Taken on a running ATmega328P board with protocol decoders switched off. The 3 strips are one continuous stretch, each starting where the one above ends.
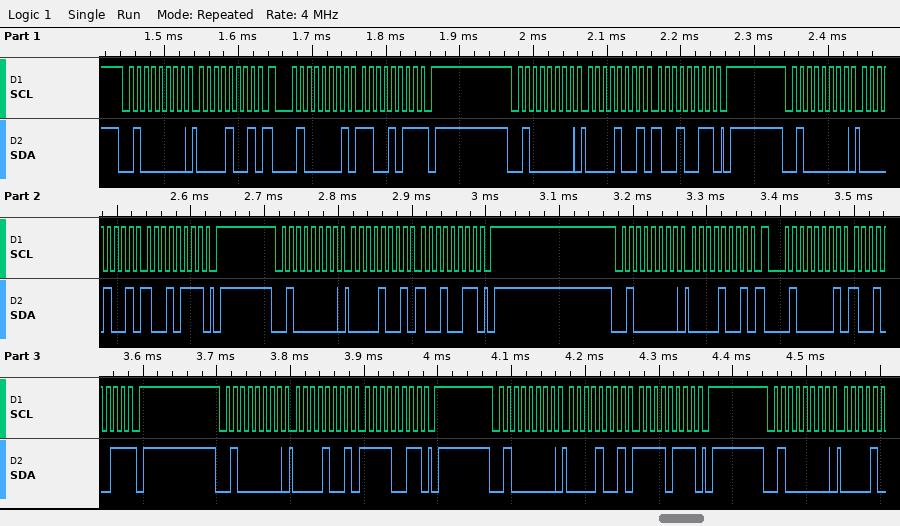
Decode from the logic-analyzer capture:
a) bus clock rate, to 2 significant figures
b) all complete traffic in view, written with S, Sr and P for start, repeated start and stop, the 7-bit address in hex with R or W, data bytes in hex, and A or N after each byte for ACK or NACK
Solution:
100 kHz
S 20W A 09 A Sr 20R A CB N P S 20W A 09 A 93 A P S 20W A 09 A 97 A P S 20W A 09 A 93 A P S 20W A 09 A Sr 20R A 93 N P S 20W A 09 A F3 A P S 20W A 09 A F7 A P S 20W A
